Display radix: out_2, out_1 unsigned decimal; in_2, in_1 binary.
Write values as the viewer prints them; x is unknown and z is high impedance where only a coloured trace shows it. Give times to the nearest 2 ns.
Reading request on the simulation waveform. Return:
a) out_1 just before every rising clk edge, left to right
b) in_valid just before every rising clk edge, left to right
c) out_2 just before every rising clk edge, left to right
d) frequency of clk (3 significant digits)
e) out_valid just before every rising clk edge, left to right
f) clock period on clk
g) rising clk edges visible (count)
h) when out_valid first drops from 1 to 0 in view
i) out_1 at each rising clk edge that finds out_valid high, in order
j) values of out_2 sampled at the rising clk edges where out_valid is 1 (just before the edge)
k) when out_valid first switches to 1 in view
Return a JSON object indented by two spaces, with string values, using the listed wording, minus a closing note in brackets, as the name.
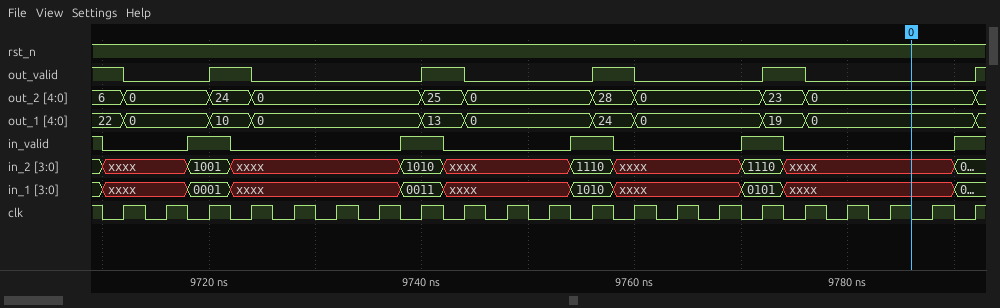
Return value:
{
  "out_1 just before every rising clk edge, left to right": "22, 0, 0, 10, 0, 0, 0, 0, 13, 0, 0, 0, 24, 0, 0, 0, 19, 0, 0, 0, 0",
  "in_valid just before every rising clk edge, left to right": "0 0 1 0 0 0 0 1 0 0 0 1 0 0 0 1 0 0 0 0 1",
  "out_2 just before every rising clk edge, left to right": "6, 0, 0, 24, 0, 0, 0, 0, 25, 0, 0, 0, 28, 0, 0, 0, 23, 0, 0, 0, 0",
  "frequency of clk": "250 MHz",
  "out_valid just before every rising clk edge, left to right": "1 0 0 1 0 0 0 0 1 0 0 0 1 0 0 0 1 0 0 0 0",
  "clock period on clk": "4 ns",
  "rising clk edges visible": "21",
  "when out_valid first drops from 1 to 0 in view": "9712 ns",
  "out_1 at each rising clk edge that finds out_valid high, in order": "22, 10, 13, 24, 19",
  "values of out_2 sampled at the rising clk edges where out_valid is 1": "6, 24, 25, 28, 23",
  "when out_valid first switches to 1 in view": "9720 ns"
}
